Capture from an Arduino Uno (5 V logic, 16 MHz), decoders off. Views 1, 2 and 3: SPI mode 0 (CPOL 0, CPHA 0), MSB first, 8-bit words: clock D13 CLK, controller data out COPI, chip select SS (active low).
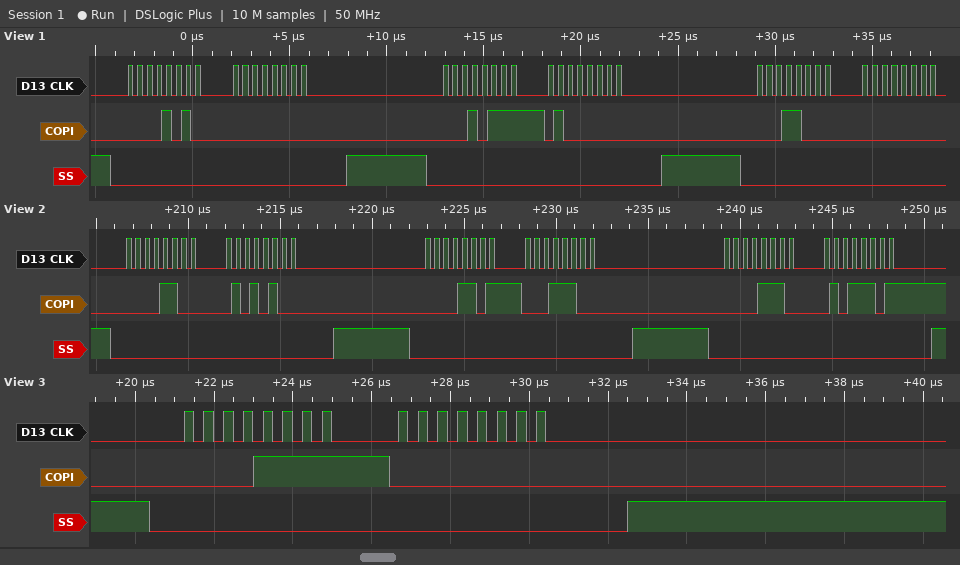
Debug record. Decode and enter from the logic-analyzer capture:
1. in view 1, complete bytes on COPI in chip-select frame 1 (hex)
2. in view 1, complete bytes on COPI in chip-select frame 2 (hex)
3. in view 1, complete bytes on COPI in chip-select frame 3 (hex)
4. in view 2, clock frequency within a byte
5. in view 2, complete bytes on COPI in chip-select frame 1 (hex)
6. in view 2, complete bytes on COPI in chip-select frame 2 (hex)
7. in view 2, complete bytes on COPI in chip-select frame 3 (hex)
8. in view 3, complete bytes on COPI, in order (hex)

0x0A 0x00
0x17 0x40
0x18 0x00
2 MHz
0C 54
0D 1C
0E 5D
0F 00
